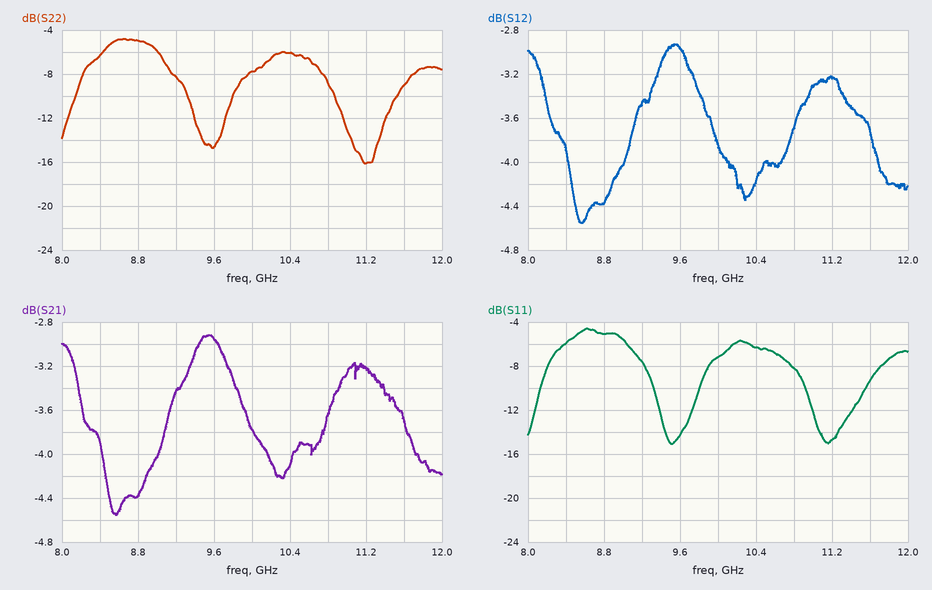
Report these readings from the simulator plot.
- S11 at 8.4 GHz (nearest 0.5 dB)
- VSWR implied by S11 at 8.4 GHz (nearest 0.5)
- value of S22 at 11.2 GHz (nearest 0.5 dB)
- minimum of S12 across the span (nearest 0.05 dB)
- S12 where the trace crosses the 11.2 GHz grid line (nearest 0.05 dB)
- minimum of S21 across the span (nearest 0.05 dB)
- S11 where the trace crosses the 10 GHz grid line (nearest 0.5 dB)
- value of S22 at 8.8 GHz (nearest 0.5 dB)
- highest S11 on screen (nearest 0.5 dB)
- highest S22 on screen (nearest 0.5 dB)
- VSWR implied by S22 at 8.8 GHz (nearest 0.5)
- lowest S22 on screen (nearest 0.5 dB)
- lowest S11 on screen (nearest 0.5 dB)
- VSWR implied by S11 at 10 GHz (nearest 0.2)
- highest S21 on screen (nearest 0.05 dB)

-6.0 dB
3.0
-16.0 dB
-4.55 dB
-3.25 dB
-4.55 dB
-7.0 dB
-5.0 dB
-4.5 dB
-5.0 dB
3.5
-16.0 dB
-15.0 dB
2.6
-2.90 dB
